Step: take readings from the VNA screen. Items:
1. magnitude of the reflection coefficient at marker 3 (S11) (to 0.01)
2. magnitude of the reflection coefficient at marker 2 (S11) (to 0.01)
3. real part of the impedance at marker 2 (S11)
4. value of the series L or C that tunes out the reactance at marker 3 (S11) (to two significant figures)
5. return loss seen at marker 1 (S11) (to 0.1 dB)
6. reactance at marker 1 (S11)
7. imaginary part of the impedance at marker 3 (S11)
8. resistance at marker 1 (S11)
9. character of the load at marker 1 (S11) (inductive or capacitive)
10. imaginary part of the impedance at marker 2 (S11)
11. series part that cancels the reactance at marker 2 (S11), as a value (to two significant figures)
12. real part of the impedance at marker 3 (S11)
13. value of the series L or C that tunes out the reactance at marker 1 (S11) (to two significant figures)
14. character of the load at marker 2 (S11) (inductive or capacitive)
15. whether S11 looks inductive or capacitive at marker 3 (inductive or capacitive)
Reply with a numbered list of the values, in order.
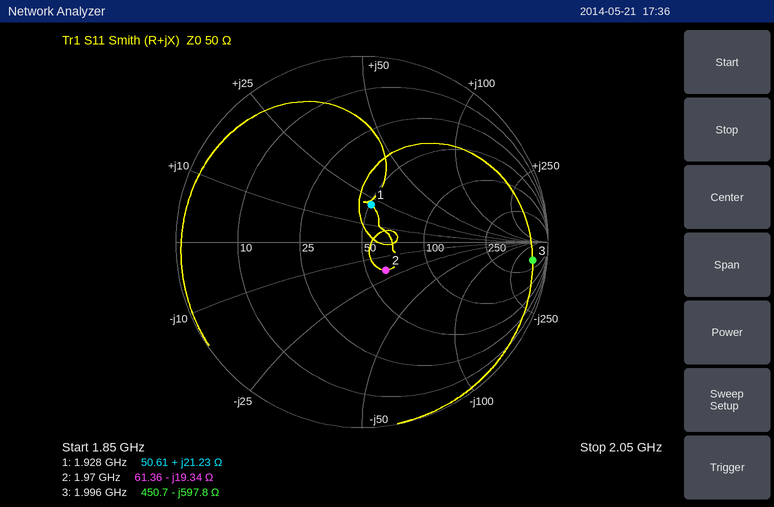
1. 0.92
2. 0.20
3. 61.36 Ω
4. 48 nH
5. 13.7 dB
6. +21.23 Ω
7. -597.8 Ω
8. 50.61 Ω
9. inductive
10. -19.34 Ω
11. 1.6 nH
12. 450.7 Ω
13. 3.9 pF
14. capacitive
15. capacitive
